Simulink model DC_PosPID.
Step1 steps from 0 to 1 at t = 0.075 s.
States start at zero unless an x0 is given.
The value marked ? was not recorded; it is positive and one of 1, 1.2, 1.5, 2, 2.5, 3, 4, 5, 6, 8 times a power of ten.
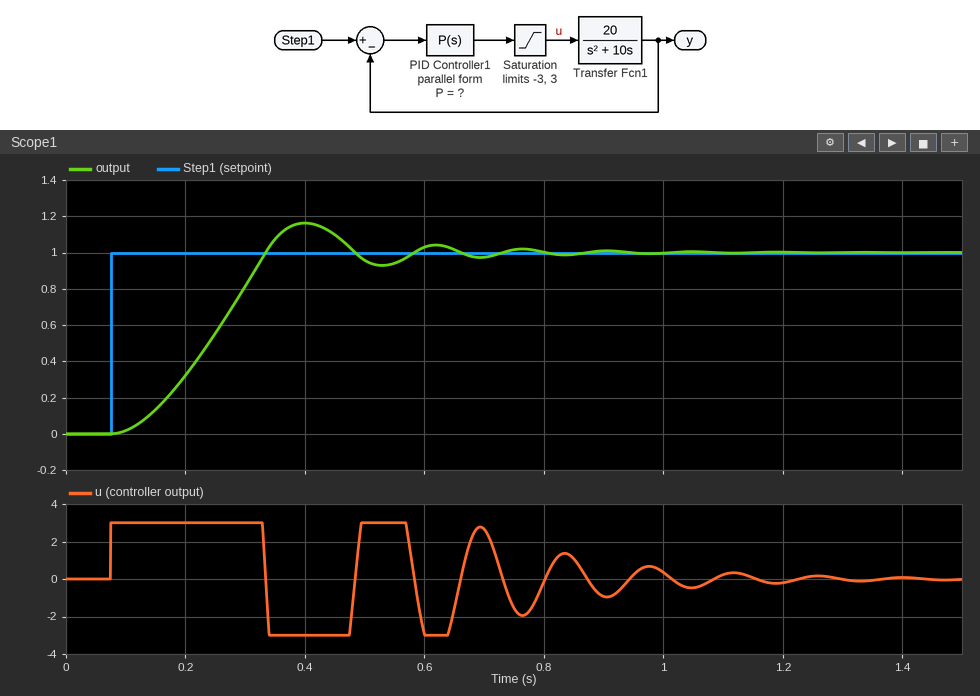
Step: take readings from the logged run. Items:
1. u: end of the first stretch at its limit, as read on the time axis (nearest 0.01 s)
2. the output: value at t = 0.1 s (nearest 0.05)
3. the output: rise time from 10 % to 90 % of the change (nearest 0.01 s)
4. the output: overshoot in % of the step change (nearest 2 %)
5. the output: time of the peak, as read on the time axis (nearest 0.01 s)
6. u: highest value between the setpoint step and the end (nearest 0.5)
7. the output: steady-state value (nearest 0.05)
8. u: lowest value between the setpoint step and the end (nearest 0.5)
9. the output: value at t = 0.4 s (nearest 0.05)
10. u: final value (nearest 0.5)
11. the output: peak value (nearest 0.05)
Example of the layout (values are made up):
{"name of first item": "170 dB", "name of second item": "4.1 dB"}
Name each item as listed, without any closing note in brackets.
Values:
{"u: end of the first stretch at its limit, as read on the time axis": "0.33 s", "the output: value at t = 0.1 s": "0.00", "the output: rise time from 10 % to 90 % of the change": "0.18 s", "the output: overshoot in % of the step change": "16 %", "the output: time of the peak, as read on the time axis": "0.40 s", "u: highest value between the setpoint step and the end": "3.0", "the output: steady-state value": "1.00", "u: lowest value between the setpoint step and the end": "-3.0", "the output: value at t = 0.4 s": "1.15", "u: final value": "0.0", "the output: peak value": "1.15"}
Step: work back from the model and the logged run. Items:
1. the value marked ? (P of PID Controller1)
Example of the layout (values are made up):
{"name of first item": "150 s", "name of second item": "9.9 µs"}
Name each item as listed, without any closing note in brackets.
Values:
{"the value marked ?": "100"}
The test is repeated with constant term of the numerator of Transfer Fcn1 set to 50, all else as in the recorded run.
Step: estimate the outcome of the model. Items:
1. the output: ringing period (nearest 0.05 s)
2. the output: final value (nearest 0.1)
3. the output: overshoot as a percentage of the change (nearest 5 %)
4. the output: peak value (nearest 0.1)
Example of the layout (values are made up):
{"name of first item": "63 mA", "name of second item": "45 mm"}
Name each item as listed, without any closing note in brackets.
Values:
{"the output: ringing period": "0.20 s", "the output: final value": "1.0", "the output: overshoot as a percentage of the change": "30 %", "the output: peak value": "1.3"}
